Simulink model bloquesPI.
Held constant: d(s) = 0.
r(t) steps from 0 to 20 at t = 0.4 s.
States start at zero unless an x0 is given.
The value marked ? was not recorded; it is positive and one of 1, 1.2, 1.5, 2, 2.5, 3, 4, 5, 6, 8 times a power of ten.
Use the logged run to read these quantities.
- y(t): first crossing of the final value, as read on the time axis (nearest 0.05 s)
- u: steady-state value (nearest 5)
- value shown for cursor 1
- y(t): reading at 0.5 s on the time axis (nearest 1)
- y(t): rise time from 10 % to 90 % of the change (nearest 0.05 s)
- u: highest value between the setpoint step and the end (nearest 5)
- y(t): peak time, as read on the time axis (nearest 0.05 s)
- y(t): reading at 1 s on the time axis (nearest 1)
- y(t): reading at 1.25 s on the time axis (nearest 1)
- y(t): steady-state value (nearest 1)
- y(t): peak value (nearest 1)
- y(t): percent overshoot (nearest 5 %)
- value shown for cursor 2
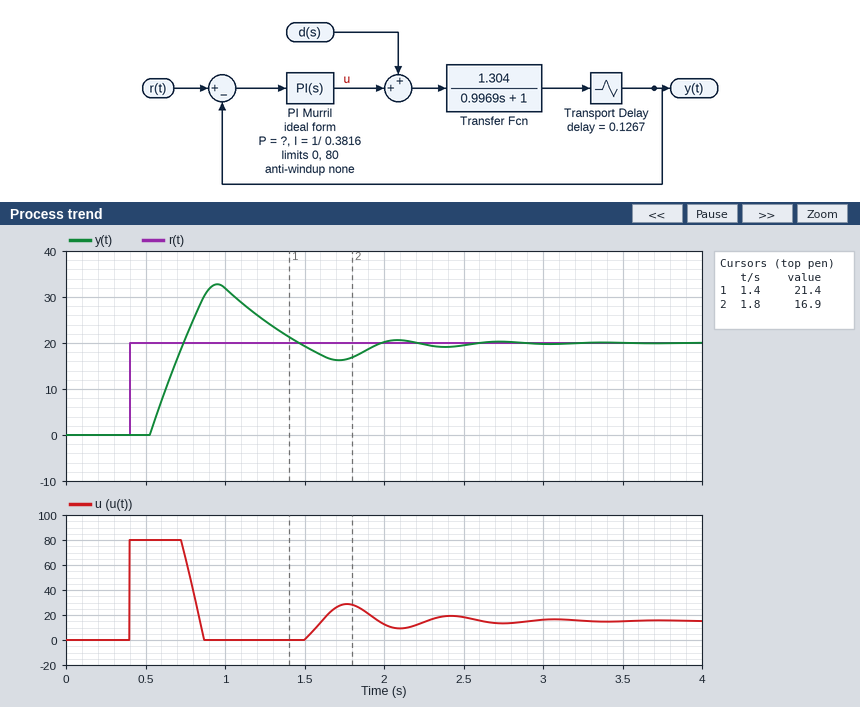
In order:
0.75 s
15
21.4
0
0.15 s
80
0.95 s
32
25
20
33
65 %
16.9
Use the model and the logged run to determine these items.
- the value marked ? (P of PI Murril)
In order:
6
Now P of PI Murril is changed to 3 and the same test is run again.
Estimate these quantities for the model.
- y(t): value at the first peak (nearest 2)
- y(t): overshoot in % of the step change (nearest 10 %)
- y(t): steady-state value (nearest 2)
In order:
26
30 %
20
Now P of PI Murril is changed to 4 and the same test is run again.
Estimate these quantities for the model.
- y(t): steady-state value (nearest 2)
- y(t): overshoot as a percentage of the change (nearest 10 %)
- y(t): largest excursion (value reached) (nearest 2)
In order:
20
50 %
30
